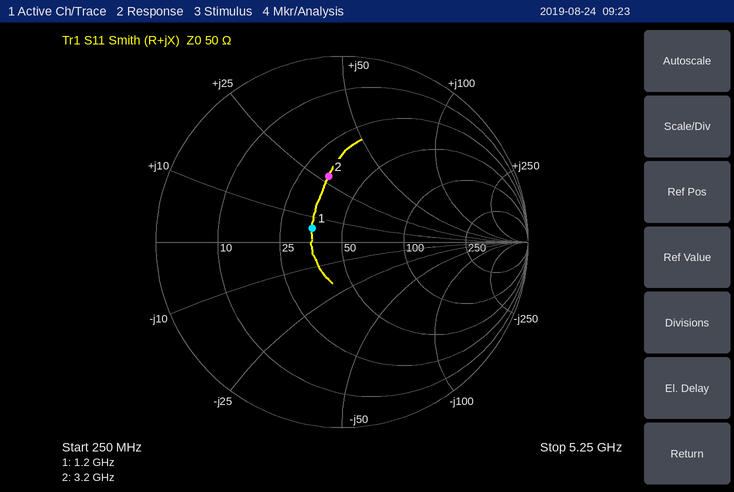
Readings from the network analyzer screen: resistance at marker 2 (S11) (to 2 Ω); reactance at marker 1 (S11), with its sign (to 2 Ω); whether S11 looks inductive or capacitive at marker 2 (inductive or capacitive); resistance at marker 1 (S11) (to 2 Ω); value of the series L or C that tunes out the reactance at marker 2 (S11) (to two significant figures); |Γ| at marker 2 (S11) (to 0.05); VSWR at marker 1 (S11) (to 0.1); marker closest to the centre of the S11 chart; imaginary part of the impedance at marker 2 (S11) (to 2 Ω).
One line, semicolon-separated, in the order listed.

34 Ω; +6 Ω; inductive; 36 Ω; 1.8 pF; 0.35; 1.4; marker 1; +28 Ω
